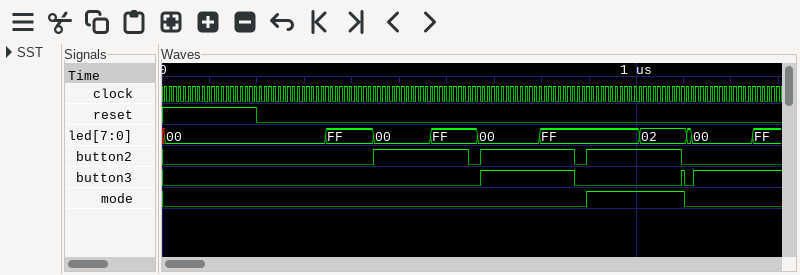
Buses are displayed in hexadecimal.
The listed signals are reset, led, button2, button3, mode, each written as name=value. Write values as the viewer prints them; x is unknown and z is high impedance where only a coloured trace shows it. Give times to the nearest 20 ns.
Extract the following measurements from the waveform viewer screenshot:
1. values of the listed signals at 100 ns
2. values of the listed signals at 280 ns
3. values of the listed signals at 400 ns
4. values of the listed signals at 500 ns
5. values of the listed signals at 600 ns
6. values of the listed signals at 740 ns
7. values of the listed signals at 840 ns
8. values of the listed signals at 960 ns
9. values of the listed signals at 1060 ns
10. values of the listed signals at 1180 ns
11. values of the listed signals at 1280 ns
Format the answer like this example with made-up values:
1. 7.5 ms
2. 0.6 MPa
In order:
1. reset=1, led=00, button2=0, button3=0, mode=0
2. reset=0, led=00, button2=0, button3=0, mode=0
3. reset=0, led=FF, button2=0, button3=0, mode=0
4. reset=0, led=00, button2=1, button3=0, mode=0
5. reset=0, led=FF, button2=1, button3=0, mode=0
6. reset=0, led=00, button2=1, button3=1, mode=0
7. reset=0, led=FF, button2=1, button3=1, mode=0
8. reset=0, led=FF, button2=1, button3=0, mode=1
9. reset=0, led=02, button2=1, button3=0, mode=1
10. reset=0, led=00, button2=0, button3=1, mode=0
11. reset=0, led=FF, button2=0, button3=1, mode=0
